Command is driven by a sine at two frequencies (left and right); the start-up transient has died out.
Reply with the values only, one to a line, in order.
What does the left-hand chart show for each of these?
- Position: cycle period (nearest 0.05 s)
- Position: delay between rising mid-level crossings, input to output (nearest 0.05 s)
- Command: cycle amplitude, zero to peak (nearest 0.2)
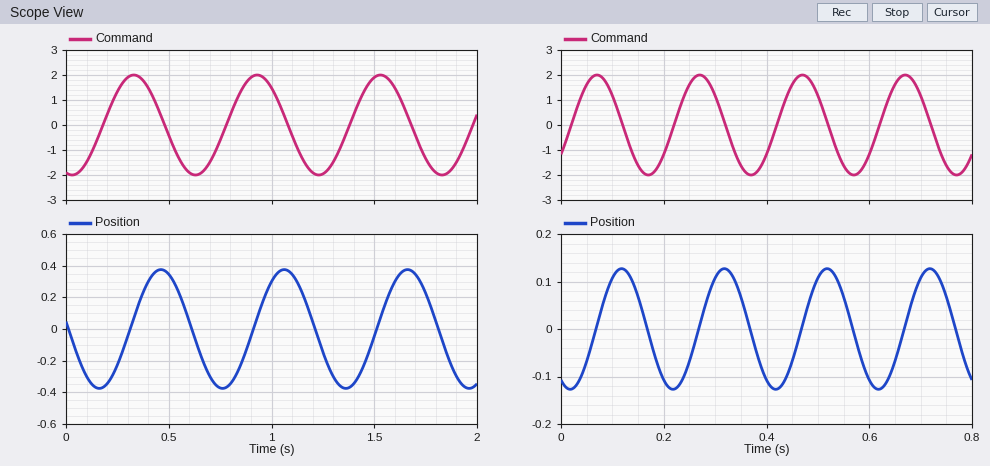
0.60 s
0.15 s
2.0
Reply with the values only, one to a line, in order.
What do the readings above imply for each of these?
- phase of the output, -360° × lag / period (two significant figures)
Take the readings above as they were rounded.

-90°
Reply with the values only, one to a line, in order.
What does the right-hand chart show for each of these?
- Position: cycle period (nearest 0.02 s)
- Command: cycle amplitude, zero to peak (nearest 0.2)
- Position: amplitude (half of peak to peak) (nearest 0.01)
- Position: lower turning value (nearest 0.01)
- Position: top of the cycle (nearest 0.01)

0.20 s
2.0
0.13
-0.13
0.13
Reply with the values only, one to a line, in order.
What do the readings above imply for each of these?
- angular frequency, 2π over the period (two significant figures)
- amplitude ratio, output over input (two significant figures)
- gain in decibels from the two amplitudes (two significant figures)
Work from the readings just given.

31 rad/s
0.065
-24 dB
